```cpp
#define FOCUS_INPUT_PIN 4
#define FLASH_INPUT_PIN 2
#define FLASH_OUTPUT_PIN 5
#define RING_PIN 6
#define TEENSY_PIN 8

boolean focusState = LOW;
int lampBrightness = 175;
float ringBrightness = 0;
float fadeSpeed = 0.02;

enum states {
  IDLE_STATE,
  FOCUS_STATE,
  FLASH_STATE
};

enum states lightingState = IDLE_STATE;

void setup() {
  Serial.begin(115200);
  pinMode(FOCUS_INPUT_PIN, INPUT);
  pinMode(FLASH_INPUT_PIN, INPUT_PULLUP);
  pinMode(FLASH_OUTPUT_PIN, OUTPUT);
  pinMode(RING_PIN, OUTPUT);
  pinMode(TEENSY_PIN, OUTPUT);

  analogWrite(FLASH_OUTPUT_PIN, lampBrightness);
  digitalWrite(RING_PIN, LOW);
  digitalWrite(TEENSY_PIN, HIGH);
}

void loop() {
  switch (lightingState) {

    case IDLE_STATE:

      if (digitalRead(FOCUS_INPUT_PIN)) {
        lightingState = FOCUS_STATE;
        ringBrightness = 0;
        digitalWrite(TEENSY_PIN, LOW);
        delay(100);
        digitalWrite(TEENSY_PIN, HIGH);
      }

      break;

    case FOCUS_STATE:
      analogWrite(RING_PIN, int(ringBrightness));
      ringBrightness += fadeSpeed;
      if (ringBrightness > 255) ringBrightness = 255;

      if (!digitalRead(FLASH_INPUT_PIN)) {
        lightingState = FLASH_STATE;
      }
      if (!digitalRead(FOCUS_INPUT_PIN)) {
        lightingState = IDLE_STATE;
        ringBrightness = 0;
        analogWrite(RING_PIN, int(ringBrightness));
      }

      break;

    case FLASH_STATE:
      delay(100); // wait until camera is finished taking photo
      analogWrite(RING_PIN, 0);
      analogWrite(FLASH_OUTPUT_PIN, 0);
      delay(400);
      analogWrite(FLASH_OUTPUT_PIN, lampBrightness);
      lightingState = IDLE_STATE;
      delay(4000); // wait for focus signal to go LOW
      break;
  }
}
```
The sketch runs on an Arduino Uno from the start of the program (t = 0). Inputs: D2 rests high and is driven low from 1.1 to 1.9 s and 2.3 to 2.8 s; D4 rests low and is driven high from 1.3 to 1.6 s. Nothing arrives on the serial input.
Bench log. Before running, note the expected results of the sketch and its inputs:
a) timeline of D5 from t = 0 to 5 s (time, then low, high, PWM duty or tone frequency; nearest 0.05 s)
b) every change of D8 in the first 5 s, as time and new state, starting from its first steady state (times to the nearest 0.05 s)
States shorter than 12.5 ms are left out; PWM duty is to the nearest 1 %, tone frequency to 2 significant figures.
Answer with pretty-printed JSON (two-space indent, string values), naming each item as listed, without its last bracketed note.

{
  "timeline of D5 from t = 0 to 5 s": "0 s PWM 69 %; 1.5 s low; 1.9 s PWM 69 %",
  "every change of D8 in the first 5 s, as time and new state, starting from its first steady state": "0 s high; 1.3 s low; 1.4 s high"
}
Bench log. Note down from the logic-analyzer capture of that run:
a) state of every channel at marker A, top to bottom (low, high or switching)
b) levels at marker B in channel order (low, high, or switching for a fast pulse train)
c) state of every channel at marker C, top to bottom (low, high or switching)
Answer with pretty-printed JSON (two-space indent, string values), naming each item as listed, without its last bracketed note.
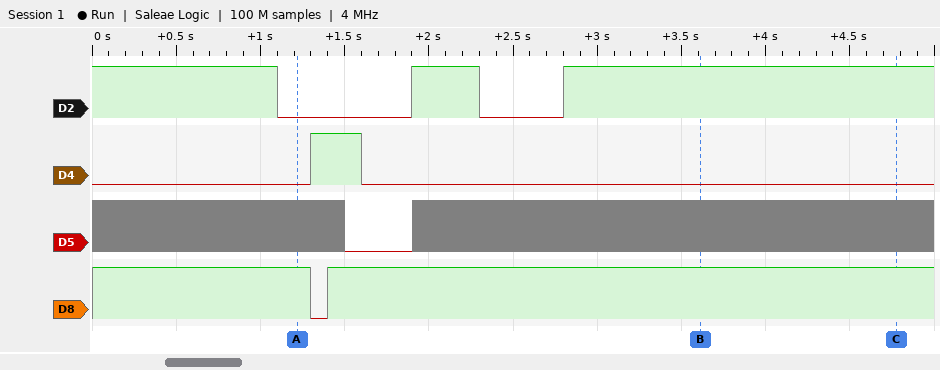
{
  "state of every channel at marker A, top to bottom": "D2 low, D4 low, D5 switching, D8 high",
  "levels at marker B in channel order": "D2 high, D4 low, D5 switching, D8 high",
  "state of every channel at marker C, top to bottom": "D2 high, D4 low, D5 switching, D8 high"
}
